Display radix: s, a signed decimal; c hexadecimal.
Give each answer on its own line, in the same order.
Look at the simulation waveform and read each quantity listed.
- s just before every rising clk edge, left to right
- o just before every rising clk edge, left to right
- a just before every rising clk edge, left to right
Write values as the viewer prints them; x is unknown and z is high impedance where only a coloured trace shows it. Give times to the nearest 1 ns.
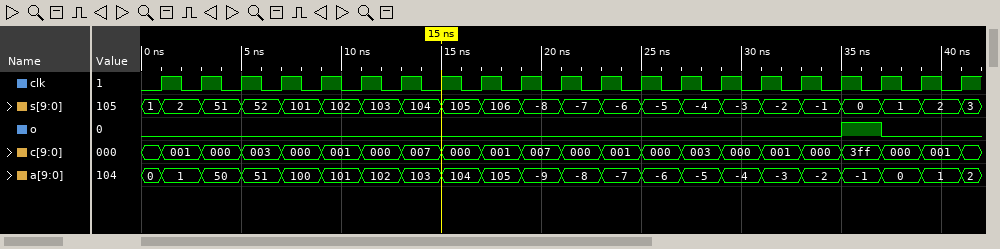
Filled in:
1, 2, 51, 52, 101, 102, 103, 104, 105, 106, -8, -7, -6, -5, -4, -3, -2, -1, 0, 1, 2
0 0 0 0 0 0 0 0 0 0 0 0 0 0 0 0 0 0 1 0 0
0, 1, 50, 51, 100, 101, 102, 103, 104, 105, -9, -8, -7, -6, -5, -4, -3, -2, -1, 0, 1
